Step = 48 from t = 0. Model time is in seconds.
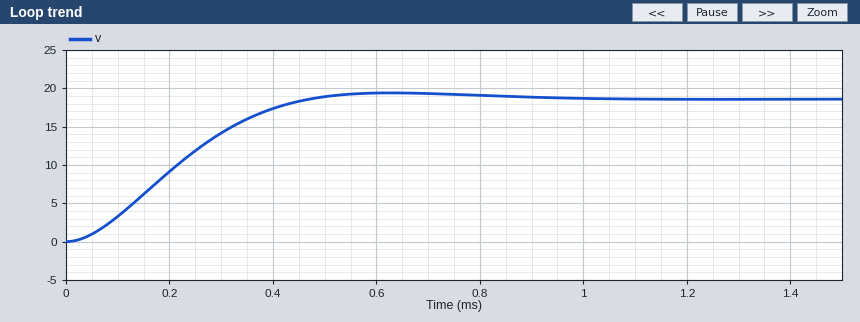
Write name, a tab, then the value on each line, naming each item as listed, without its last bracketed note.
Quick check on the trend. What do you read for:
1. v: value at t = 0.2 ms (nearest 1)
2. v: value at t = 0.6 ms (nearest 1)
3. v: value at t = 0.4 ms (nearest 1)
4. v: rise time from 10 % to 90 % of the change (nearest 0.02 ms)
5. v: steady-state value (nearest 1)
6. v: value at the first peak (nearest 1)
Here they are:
v: value at t = 0.2 ms	9
v: value at t = 0.6 ms	19
v: value at t = 0.4 ms	17
v: rise time from 10 % to 90 % of the change	0.30 ms
v: steady-state value	19
v: value at the first peak	19
